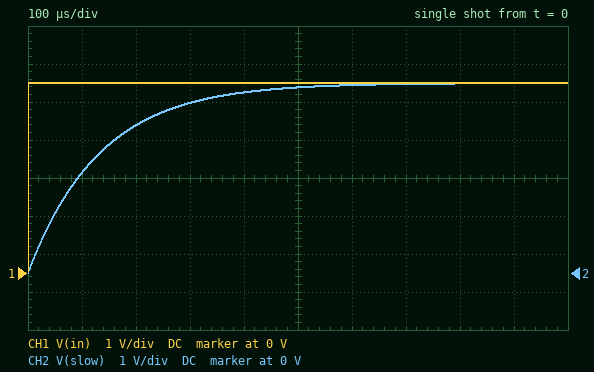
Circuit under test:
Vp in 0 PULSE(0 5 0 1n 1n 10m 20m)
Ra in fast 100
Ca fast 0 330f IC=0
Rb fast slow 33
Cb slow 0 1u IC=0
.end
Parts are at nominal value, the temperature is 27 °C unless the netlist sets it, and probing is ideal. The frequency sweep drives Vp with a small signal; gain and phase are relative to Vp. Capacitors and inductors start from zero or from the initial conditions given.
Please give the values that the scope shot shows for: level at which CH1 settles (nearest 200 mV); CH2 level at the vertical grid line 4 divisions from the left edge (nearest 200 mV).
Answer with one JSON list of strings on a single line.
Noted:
["5.0 V", "4.8 V"]
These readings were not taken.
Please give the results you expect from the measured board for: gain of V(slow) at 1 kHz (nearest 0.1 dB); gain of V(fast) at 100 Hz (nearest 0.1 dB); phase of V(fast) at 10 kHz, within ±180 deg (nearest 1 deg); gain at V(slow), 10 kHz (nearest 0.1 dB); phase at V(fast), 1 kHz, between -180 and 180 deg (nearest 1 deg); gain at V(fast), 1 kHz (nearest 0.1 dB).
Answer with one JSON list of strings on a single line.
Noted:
["-2.3 dB", "0 dB", "-19 deg", "-18.5 dB", "-28 deg", "-2.1 dB"]
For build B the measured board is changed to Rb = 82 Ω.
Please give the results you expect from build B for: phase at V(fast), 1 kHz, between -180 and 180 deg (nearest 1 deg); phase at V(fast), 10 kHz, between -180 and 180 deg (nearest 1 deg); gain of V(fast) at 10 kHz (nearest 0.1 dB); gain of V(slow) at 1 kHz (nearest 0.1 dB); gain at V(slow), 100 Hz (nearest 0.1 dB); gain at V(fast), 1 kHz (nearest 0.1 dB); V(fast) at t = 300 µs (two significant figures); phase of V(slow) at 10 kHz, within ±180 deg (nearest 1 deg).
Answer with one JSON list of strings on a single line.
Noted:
["-22 deg", "-6 deg", "-6.8 dB", "-3.6 dB", "-0.1 dB", "-2.6 dB", "4.5 V", "-85 deg"]
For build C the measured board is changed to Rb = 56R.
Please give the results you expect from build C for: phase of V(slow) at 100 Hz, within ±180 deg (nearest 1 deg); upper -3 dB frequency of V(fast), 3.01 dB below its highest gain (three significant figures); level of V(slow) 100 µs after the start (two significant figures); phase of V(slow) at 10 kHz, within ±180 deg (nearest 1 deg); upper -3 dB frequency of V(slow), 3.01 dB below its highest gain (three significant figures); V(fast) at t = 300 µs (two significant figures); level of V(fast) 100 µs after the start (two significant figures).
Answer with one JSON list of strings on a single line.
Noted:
["-6 deg", "1.18 kHz", "2.4 V", "-84 deg", "1.02 kHz", "4.5 V", "3.3 V"]
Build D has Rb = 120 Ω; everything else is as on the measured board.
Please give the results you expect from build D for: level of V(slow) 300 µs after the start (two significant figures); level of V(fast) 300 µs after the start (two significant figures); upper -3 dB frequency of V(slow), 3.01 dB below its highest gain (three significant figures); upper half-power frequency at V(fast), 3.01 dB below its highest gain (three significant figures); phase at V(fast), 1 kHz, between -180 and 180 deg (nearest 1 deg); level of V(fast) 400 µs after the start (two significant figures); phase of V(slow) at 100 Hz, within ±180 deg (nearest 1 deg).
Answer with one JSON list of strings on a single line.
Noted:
["3.7 V", "4.4 V", "723 Hz", "1.14 kHz", "-17 deg", "4.6 V", "-8 deg"]
